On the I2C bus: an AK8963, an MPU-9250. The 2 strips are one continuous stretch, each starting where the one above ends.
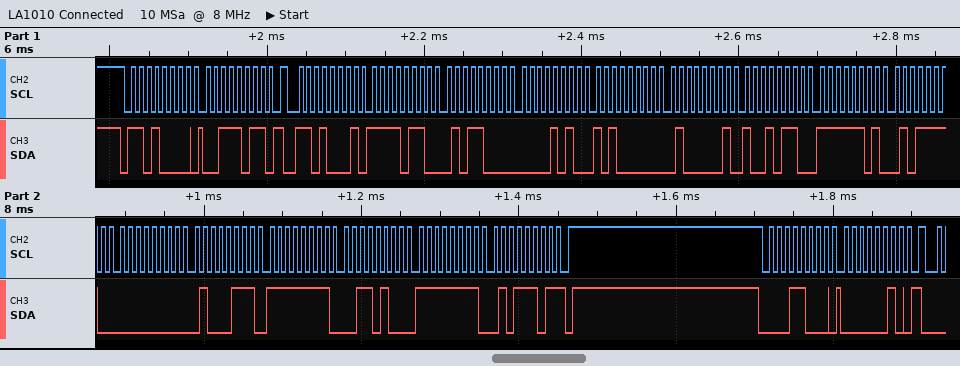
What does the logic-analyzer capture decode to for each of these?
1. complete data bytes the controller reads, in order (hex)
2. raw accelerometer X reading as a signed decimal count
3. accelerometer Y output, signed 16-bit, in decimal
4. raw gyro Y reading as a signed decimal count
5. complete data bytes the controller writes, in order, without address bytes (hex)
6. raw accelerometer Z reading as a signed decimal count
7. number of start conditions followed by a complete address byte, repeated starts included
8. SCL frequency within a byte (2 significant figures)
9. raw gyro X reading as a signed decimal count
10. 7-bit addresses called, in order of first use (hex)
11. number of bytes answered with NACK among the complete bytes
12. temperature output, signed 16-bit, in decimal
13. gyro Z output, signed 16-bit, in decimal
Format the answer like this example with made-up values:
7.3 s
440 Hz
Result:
F6 58 0A A0 41 96 FD 5E 00 47 FF 34 FF 5D
-2472
2720
-204
3B 02
16790
3
100 kHz
71
0x68 0x0C
1
-674
-163
